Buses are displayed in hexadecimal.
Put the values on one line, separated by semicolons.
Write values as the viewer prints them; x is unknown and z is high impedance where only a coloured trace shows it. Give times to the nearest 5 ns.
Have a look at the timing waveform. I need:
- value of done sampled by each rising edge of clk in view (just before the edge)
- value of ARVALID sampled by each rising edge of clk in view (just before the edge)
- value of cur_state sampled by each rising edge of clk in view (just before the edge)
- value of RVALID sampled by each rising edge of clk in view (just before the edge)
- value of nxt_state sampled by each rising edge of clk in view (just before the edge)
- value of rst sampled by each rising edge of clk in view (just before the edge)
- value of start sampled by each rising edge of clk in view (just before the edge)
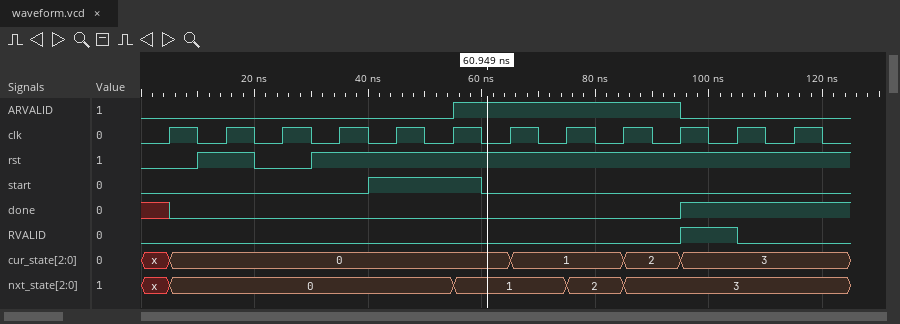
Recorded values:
x 0 0 0 0 0 0 0 0 0 1 1; 0 0 0 0 0 0 1 1 1 1 0 0; x, 0, 0, 0, 0, 0, 0, 1, 1, 2, 3, 3; 0 0 0 0 0 0 0 0 0 0 1 0; x, 0, 0, 0, 0, 0, 1, 1, 2, 3, 3, 3; 0 1 0 1 1 1 1 1 1 1 1 1; 0 0 0 0 1 1 0 0 0 0 0 0
